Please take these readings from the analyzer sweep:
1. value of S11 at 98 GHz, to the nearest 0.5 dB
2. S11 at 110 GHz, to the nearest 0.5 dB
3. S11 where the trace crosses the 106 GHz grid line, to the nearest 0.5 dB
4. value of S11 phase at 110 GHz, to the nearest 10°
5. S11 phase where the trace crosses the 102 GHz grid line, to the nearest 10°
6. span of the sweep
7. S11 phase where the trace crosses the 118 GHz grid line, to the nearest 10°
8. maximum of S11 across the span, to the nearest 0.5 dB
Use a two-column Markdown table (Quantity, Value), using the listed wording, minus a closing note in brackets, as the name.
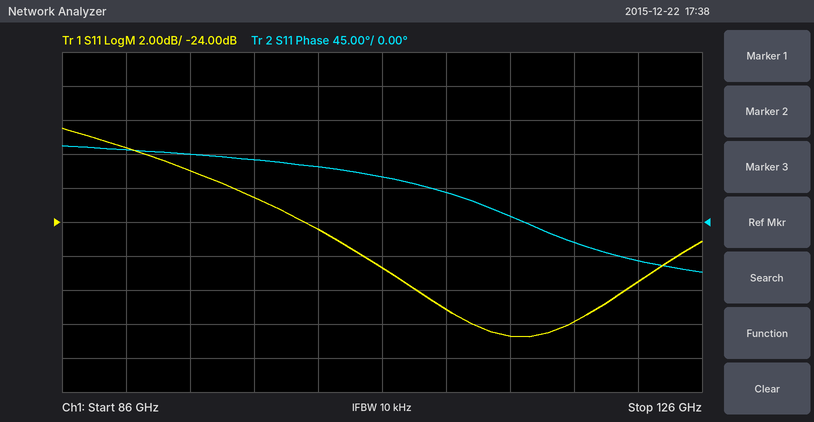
| Quantity | Value |
|---|---|
| value of S11 at 98 GHz, to the nearest 0.5 dB | -22.5 dB |
| S11 at 110 GHz, to the nearest 0.5 dB | -29.0 dB |
| S11 where the trace crosses the 106 GHz grid line, to the nearest 0.5 dB | -26.5 dB |
| value of S11 phase at 110 GHz, to the nearest 10° | 40° |
| S11 phase where the trace crosses the 102 GHz grid line, to the nearest 10° | 70° |
| span of the sweep | 40 GHz |
| S11 phase where the trace crosses the 118 GHz grid line, to the nearest 10° | -30° |
| maximum of S11 across the span, to the nearest 0.5 dB | -18.5 dB |
